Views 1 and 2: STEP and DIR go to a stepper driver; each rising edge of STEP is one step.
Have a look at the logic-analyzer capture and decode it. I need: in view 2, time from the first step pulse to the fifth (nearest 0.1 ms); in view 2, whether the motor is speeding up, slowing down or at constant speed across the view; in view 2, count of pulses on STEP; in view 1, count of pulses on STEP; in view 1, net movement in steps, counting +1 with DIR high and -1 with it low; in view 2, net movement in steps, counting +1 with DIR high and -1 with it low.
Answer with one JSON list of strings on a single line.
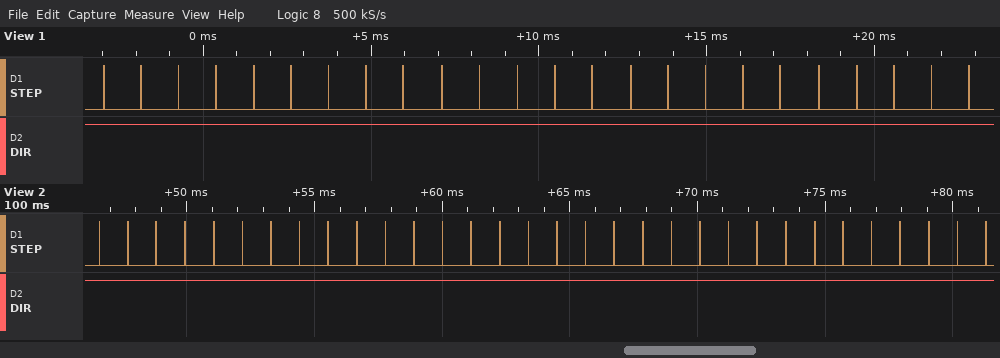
["4.5 ms", "constant speed", "32", "24", "+24", "+32"]
